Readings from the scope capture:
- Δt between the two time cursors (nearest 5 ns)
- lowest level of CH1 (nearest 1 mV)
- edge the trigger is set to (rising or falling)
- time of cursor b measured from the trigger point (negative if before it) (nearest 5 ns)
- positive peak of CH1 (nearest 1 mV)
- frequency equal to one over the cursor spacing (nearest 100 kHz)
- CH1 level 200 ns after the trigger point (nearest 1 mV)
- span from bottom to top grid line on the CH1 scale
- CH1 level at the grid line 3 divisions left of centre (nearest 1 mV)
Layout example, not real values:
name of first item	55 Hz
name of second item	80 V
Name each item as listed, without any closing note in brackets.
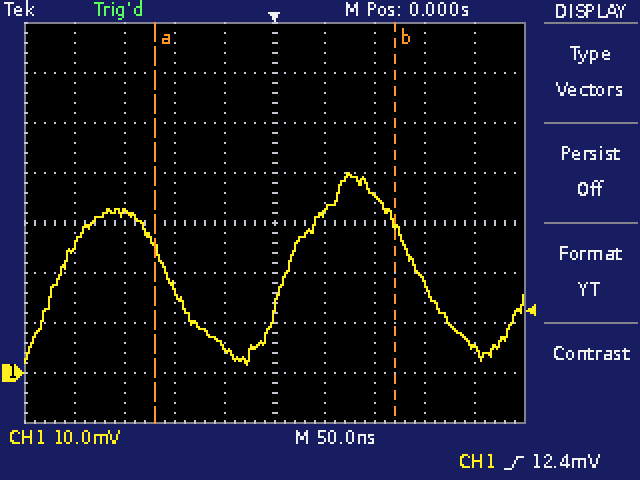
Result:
Δt between the two time cursors	240 ns
lowest level of CH1	2 mV
edge the trigger is set to	rising
time of cursor b measured from the trigger point (negative if before it)	+120 ns
positive peak of CH1	40 mV
frequency equal to one over the cursor spacing	4.2 MHz
CH1 level 200 ns after the trigger point	5 mV
span from bottom to top grid line on the CH1 scale	80 mV
CH1 level at the grid line 3 divisions left of centre	32 mV
